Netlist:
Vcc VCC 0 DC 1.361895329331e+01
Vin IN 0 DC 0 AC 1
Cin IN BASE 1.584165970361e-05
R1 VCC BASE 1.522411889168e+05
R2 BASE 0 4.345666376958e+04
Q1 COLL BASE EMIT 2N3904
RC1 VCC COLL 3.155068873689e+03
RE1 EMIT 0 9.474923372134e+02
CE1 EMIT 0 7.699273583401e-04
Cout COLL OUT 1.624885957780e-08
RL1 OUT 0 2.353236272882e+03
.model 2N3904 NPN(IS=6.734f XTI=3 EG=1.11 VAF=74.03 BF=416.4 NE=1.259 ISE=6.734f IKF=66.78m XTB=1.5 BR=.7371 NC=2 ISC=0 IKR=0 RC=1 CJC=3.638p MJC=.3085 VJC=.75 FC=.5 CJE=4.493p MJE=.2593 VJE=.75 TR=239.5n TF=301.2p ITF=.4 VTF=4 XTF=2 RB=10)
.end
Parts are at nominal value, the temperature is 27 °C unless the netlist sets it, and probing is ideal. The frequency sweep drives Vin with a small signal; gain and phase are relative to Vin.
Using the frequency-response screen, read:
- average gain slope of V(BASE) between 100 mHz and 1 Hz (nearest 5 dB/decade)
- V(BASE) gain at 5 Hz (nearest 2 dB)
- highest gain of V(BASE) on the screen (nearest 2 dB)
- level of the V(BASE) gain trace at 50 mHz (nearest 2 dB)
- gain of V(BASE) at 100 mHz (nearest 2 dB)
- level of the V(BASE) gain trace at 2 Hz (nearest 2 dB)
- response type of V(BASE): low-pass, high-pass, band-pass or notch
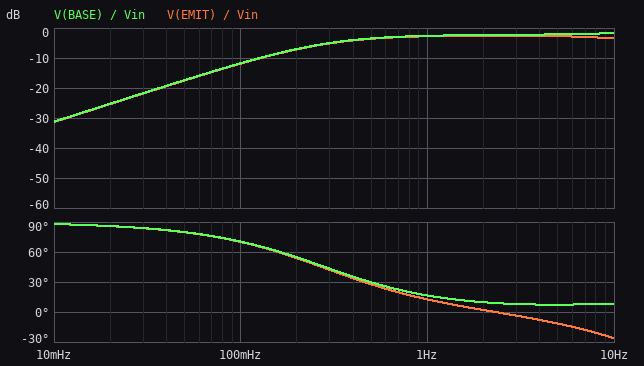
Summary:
10 dB/decade
-2 dB
-2 dB
-18 dB
-12 dB
-2 dB
high-pass
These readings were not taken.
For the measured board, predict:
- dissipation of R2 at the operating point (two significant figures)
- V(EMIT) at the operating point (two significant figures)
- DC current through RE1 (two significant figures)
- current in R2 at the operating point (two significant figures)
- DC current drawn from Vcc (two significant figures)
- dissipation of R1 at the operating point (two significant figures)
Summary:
150 µW
1.9 V
2.0 mA
59 µA
2.1 mA
800 µW
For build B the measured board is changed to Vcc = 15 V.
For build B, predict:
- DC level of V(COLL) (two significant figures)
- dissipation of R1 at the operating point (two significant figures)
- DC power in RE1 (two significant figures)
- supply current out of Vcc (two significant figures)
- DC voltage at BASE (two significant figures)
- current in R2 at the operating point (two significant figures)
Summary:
7.9 V
970 µW
4.9 mW
2.3 mA
2.8 V
65 µA
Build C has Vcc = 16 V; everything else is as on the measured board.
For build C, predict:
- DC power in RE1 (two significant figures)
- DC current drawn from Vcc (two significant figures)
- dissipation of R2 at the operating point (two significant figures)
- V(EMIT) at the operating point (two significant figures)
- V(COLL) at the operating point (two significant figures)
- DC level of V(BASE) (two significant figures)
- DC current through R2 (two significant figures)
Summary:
5.8 mW
2.5 mA
210 µW
2.3 V
8.3 V
3.0 V
70 µA
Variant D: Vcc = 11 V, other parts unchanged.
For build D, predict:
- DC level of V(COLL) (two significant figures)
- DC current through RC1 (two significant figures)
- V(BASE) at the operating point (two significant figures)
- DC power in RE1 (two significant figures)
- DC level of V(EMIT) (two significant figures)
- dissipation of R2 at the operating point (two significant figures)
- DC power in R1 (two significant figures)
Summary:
6.3 V
1.5 mA
2.1 V
2.1 mW
1.4 V
100 µW
520 µW
